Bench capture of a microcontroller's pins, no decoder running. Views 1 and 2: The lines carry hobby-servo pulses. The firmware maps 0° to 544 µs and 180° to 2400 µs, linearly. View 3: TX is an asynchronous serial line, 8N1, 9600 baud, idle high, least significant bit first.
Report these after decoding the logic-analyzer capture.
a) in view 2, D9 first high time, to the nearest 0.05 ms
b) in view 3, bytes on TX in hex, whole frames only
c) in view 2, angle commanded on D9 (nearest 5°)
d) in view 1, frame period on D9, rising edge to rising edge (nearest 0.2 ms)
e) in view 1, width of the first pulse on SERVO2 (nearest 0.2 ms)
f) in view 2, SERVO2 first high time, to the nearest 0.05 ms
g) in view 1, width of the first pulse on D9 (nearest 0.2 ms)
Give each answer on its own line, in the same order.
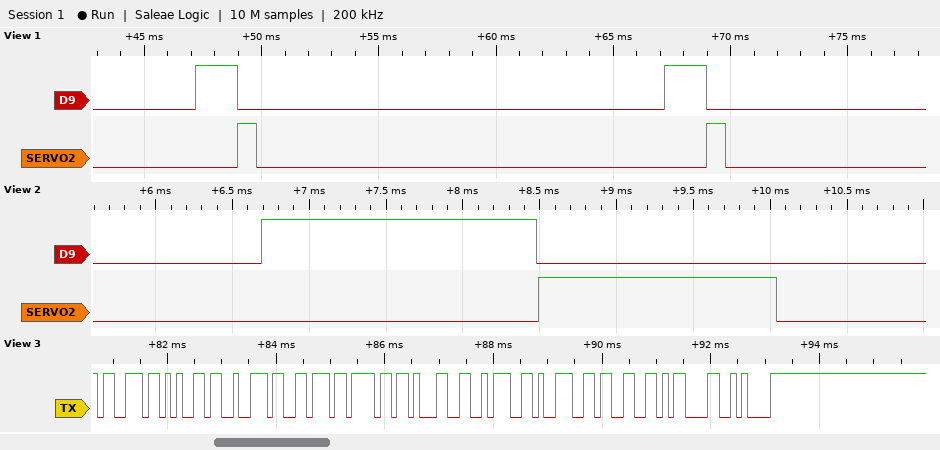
1.80 ms
73 65 72 76 6F 31 3A 39 33 0D 0A
120°
20.0 ms
0.8 ms
1.55 ms
1.8 ms
